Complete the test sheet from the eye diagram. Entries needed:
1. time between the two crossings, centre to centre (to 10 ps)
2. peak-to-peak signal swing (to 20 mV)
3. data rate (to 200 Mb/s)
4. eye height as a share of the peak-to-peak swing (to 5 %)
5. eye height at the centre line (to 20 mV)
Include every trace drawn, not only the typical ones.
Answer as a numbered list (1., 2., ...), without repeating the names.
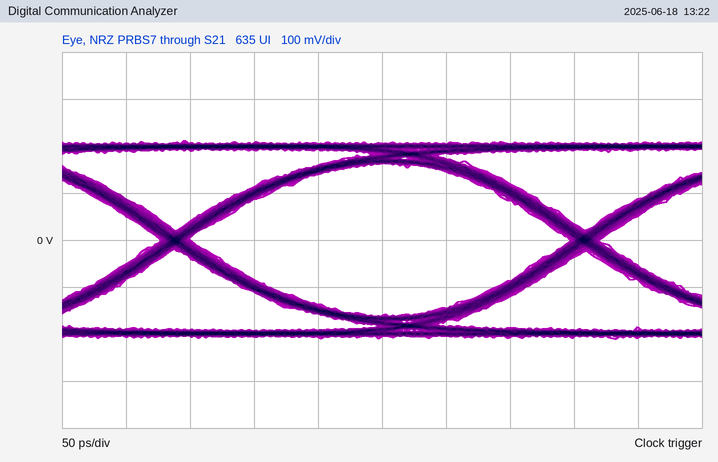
1. 320 ps
2. 420 mV
3. 3.2 Gb/s
4. 75 %
5. 320 mV
